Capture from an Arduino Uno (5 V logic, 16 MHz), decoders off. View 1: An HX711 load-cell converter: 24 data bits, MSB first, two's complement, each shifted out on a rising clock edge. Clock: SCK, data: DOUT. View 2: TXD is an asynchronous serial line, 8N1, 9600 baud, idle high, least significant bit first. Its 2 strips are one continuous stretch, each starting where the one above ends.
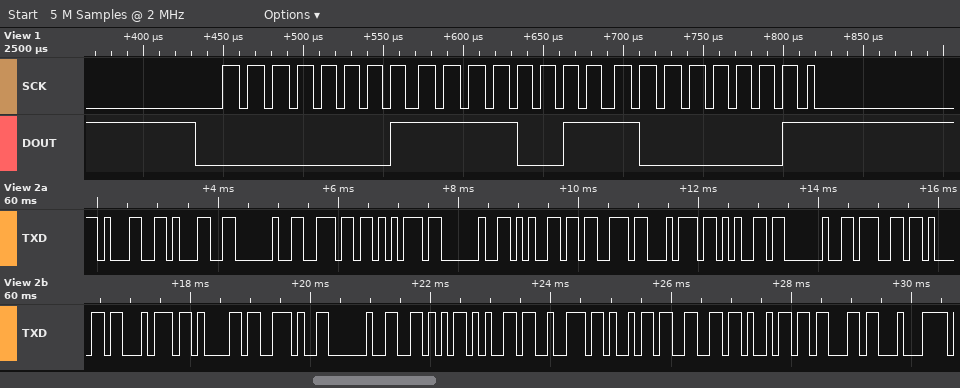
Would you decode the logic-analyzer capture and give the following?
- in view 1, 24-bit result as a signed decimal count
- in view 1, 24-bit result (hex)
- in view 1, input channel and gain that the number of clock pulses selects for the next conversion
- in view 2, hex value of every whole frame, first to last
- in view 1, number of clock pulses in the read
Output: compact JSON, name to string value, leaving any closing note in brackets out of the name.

{"in view 1, 24-bit result as a signed decimal count": "127873", "in view 1, 24-bit result": "0x01F381", "in view 1, input channel and gain that the number of clock pulses selects for the next conversion": "channel A, gain 128", "in view 2, hex value of every whole frame, first to last": "31 31 20 6E 75 20 65 73 74 65 20 67 61 74 61 2E 20 56 65 72 69 66 69 63 C4", "in view 1, number of clock pulses in the read": "25"}
